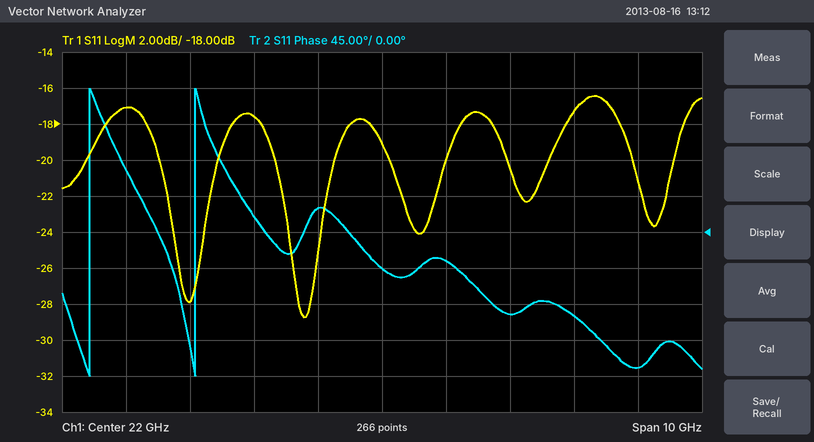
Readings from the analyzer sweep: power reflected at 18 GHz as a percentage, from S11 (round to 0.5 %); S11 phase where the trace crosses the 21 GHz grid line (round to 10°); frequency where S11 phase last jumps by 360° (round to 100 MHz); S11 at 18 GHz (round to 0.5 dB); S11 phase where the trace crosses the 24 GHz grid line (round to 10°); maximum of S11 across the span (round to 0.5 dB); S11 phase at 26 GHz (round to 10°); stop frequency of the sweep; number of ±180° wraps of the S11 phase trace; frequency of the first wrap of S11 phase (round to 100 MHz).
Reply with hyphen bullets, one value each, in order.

- 2.0 %
- 30°
- 19.1 GHz
- -17.0 dB
- -100°
- -16.5 dB
- -170°
- 27 GHz
- 2
- 17.4 GHz
